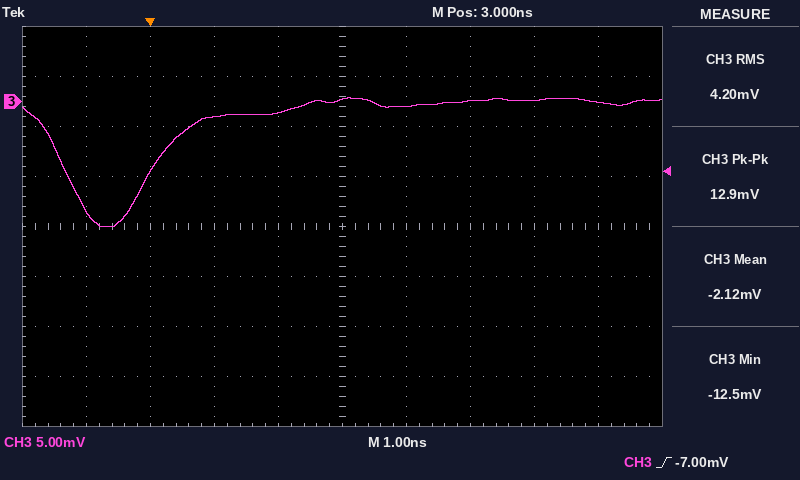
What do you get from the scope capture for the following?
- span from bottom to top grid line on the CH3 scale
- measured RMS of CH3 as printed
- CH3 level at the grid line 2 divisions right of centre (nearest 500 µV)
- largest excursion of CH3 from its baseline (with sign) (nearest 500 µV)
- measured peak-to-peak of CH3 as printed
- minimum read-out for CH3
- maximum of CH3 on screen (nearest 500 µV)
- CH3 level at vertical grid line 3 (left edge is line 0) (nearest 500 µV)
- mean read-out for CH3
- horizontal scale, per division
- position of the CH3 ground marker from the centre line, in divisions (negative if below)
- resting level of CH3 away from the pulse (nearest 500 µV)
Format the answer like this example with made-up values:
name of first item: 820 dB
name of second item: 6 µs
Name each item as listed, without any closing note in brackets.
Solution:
span from bottom to top grid line on the CH3 scale: 40 mV
measured RMS of CH3 as printed: 4.20 mV
CH3 level at the grid line 2 divisions right of centre: 0.0 mV
largest excursion of CH3 from its baseline (with sign): -12.5 mV
measured peak-to-peak of CH3 as printed: 12.9 mV
minimum read-out for CH3: -12.5 mV
maximum of CH3 on screen: 500 µV
CH3 level at vertical grid line 3 (left edge is line 0): -1.5 mV
mean read-out for CH3: -2.12 mV
horizontal scale, per division: 1 ns
position of the CH3 ground marker from the centre line, in divisions: +2.5 div
resting level of CH3 away from the pulse: 0.0 mV
